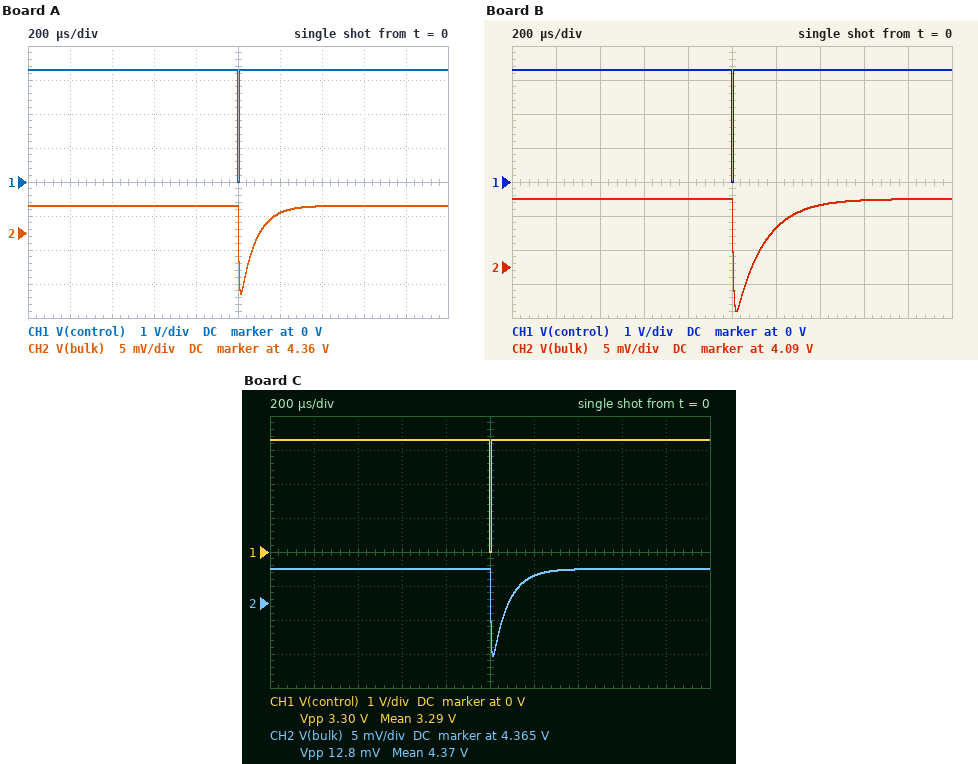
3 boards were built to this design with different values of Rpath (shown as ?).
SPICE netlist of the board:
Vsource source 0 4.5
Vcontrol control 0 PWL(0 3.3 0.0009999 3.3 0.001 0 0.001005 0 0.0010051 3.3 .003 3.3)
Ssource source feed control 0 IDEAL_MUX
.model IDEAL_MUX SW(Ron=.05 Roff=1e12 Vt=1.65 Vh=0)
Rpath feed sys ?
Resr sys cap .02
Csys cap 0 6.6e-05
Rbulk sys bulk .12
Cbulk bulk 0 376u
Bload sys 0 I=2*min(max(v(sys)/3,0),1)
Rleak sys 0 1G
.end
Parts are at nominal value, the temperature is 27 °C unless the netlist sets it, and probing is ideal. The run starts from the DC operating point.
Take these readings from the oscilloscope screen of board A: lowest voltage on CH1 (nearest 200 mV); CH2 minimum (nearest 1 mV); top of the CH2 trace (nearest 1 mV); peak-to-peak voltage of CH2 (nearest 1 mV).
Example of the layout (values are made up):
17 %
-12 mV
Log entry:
0 V
4.351 V
4.364 V
13 mV
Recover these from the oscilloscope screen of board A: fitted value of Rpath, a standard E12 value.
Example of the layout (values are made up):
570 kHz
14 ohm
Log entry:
0.018 Ω
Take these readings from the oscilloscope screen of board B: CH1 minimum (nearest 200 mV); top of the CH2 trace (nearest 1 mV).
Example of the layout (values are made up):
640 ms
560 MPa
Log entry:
0 V
4.100 V
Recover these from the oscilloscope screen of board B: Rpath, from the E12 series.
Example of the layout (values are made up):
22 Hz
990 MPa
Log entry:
0.15 Ω
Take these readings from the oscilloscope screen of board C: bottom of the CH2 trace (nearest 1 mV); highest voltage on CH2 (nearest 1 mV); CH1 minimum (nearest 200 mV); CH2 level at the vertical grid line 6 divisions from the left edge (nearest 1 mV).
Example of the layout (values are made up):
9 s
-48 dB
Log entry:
4.357 V
4.370 V
0 V
4.369 V
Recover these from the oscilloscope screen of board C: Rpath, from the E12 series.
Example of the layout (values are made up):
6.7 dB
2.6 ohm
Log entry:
0.015 Ω
